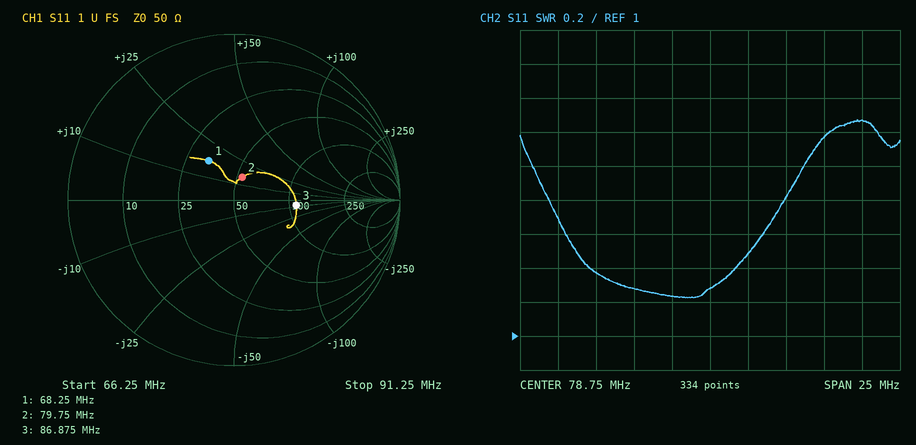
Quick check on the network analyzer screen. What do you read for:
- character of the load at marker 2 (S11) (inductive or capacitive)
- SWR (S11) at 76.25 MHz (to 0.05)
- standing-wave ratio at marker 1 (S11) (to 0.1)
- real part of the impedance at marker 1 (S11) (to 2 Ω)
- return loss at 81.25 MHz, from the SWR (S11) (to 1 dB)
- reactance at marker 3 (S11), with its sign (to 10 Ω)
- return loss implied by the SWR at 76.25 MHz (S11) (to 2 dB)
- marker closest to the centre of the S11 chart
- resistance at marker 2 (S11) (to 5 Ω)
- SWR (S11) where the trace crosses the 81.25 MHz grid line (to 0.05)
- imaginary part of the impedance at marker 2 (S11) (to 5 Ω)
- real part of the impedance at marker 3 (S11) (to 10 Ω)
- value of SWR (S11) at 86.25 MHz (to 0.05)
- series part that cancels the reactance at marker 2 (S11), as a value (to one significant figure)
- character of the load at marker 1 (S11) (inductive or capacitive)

inductive
1.25
1.8
34 Ω
14 dB
-10 Ω
20 dB
marker 2
55 Ω
1.50
+15 Ω
110 Ω
2.15
100 pF
inductive
